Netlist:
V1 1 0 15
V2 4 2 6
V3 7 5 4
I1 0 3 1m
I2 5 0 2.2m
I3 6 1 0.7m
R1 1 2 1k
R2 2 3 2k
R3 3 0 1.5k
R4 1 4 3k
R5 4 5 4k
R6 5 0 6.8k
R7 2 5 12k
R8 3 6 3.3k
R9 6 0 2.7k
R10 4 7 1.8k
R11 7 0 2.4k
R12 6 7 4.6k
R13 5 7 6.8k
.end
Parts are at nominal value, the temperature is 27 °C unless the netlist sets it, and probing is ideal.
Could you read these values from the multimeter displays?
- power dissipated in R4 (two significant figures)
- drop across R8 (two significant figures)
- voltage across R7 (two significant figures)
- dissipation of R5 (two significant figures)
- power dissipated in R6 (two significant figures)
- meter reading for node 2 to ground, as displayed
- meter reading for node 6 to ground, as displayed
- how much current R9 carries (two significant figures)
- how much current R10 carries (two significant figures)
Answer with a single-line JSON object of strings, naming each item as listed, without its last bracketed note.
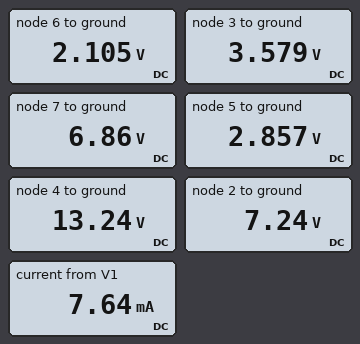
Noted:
{"power dissipated in R4": "1.0 mW", "drop across R8": "1.5 V", "voltage across R7": "4.4 V", "dissipation of R5": "27 mW", "power dissipated in R6": "1.2 mW", "meter reading for node 2 to ground, as displayed": "7.24 V", "meter reading for node 6 to ground, as displayed": "2.105 V", "how much current R9 carries": "780 µA", "how much current R10 carries": "3.5 mA"}
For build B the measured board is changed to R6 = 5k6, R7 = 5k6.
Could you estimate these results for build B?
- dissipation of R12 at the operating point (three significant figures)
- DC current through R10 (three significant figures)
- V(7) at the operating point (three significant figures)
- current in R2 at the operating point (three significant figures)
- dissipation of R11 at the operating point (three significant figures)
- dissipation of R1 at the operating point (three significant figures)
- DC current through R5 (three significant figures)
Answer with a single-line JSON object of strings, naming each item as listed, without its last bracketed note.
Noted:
{"dissipation of R12 at the operating point": "5.13 mW", "DC current through R10": "3.42 mA", "V(7) at the operating point": "6.98 V", "current in R2 at the operating point": "1.79 mA", "dissipation of R11 at the operating point": "20.3 mW", "dissipation of R1 at the operating point": "61.9 mW", "DC current through R5": "2.54 mA"}
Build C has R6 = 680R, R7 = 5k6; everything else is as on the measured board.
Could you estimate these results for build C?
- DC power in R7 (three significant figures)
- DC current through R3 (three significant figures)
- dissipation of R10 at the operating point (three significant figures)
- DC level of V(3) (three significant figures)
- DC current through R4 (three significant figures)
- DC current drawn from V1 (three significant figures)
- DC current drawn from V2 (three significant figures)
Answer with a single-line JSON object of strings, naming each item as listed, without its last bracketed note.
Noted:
{"DC power in R7": "4.55 mW", "DC current through R3": "2.17 mA", "dissipation of R10 at the operating point": "27.6 mW", "DC level of V(3)": "3.26 V", "DC current through R4": "809 µA", "DC current drawn from V1": "8.54 mA", "DC current drawn from V2": "5.87 mA"}
